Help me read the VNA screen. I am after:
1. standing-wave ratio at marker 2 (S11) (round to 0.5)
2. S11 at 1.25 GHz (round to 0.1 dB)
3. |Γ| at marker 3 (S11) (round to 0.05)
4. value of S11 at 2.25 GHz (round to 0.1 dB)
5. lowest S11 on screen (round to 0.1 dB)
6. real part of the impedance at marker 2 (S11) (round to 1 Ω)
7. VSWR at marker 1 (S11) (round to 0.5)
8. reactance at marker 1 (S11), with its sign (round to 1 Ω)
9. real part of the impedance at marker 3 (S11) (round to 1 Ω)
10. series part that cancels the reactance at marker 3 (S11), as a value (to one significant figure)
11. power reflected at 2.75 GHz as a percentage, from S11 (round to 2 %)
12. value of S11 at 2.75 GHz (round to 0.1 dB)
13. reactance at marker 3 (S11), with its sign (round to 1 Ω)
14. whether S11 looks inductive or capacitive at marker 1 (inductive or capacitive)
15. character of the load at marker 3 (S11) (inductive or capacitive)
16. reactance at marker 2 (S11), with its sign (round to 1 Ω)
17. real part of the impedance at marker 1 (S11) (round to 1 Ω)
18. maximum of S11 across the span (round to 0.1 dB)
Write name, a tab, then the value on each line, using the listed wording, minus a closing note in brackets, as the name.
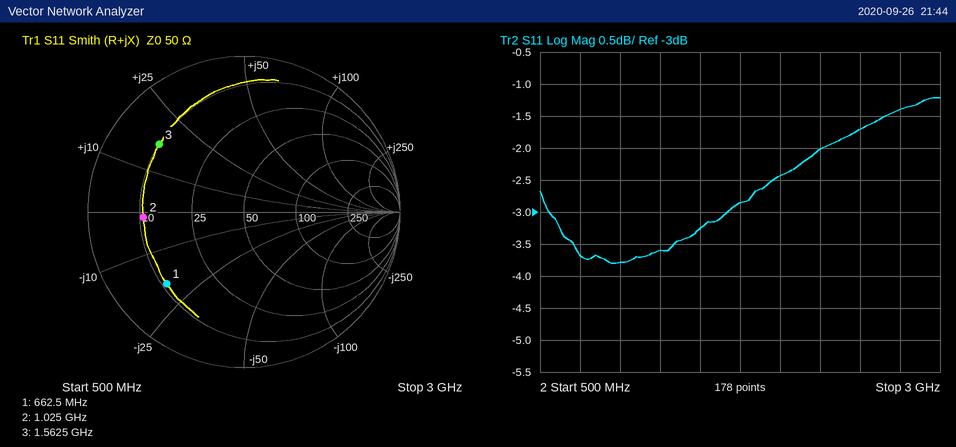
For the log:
standing-wave ratio at marker 2 (S11)	4.5
S11 at 1.25 GHz	-3.6 dB
|Γ| at marker 3 (S11)	0.70
value of S11 at 2.25 GHz	-2.0 dB
lowest S11 on screen	-3.8 dB
real part of the impedance at marker 2 (S11)	11 Ω
VSWR at marker 1 (S11)	5.0
reactance at marker 1 (S11), with its sign	-19 Ω
real part of the impedance at marker 3 (S11)	10 Ω
series part that cancels the reactance at marker 3 (S11), as a value	6 pF
power reflected at 2.75 GHz as a percentage, from S11	72 %
value of S11 at 2.75 GHz	-1.4 dB
reactance at marker 3 (S11), with its sign	+17 Ω
whether S11 looks inductive or capacitive at marker 1	capacitive
character of the load at marker 3 (S11)	inductive
reactance at marker 2 (S11), with its sign	-1 Ω
real part of the impedance at marker 1 (S11)	11 Ω
maximum of S11 across the span	-1.2 dB
